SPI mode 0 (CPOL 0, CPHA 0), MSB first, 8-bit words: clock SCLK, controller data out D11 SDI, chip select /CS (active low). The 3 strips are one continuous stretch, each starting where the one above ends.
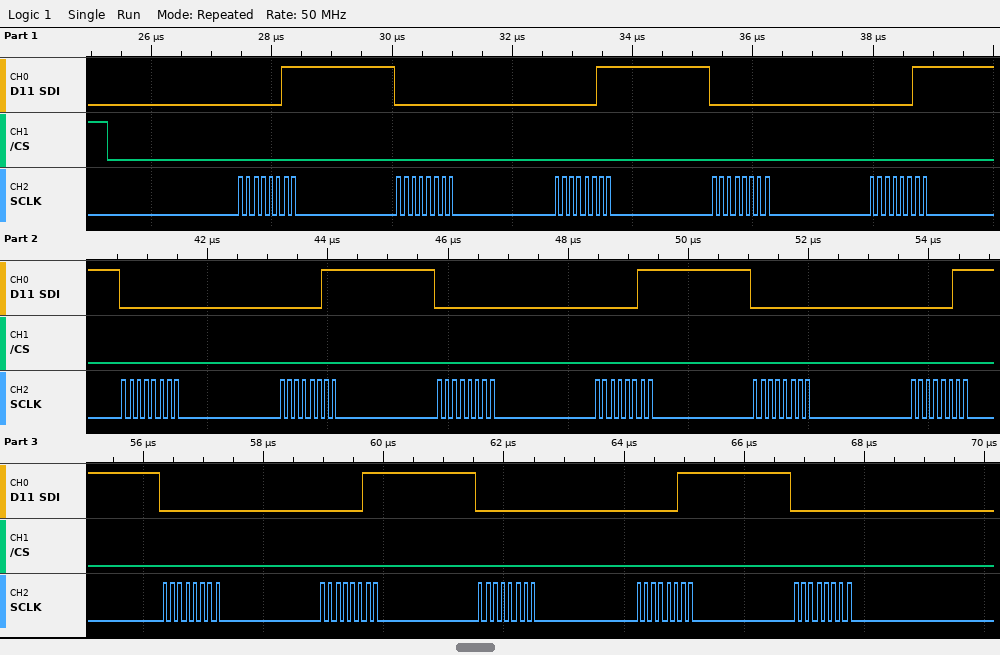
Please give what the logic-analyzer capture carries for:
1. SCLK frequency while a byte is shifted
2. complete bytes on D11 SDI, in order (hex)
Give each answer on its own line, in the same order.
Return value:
8 MHz
0x03 0x00 0x03 0x00 0x03 0x00 0x03 0x00 0x03 0x00 0x03 0x00 0x03 0x00 0x03 0x00
